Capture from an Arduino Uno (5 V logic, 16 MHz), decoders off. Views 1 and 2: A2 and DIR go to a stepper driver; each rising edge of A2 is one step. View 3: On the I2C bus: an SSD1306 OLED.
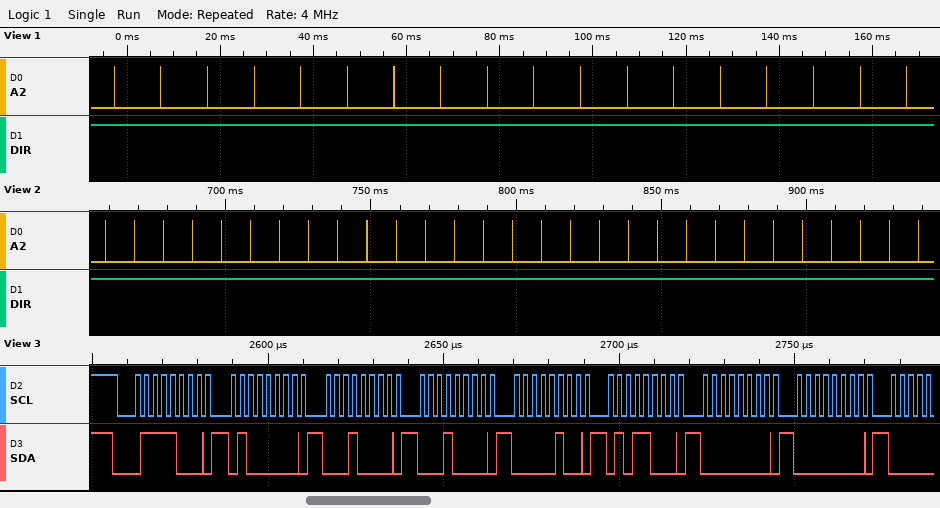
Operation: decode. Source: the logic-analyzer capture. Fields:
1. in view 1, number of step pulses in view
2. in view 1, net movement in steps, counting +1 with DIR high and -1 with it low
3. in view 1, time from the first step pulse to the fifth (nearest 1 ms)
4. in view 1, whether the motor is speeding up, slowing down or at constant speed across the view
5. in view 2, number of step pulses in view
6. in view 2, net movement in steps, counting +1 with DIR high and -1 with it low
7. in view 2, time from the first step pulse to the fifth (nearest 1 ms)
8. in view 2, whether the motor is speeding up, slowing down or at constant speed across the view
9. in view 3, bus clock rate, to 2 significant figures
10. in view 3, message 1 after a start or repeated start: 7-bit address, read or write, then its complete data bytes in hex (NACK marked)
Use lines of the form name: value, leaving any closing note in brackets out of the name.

in view 1, number of step pulses in view: 18
in view 1, net movement in steps, counting +1 with DIR high and -1 with it low: +18
in view 1, time from the first step pulse to the fifth: 40 ms
in view 1, whether the motor is speeding up, slowing down or at constant speed across the view: constant speed
in view 2, number of step pulses in view: 29
in view 2, net movement in steps, counting +1 with DIR high and -1 with it low: +29
in view 2, time from the first step pulse to the fifth: 40 ms
in view 2, whether the motor is speeding up, slowing down or at constant speed across the view: constant speed
in view 3, bus clock rate, to 2 significant figures: 400 kHz
in view 3, message 1 after a start or repeated start: 7-bit address, read or write, then its complete data bytes in hex: 0x3C write: 40 10 10 04 58 00 00
